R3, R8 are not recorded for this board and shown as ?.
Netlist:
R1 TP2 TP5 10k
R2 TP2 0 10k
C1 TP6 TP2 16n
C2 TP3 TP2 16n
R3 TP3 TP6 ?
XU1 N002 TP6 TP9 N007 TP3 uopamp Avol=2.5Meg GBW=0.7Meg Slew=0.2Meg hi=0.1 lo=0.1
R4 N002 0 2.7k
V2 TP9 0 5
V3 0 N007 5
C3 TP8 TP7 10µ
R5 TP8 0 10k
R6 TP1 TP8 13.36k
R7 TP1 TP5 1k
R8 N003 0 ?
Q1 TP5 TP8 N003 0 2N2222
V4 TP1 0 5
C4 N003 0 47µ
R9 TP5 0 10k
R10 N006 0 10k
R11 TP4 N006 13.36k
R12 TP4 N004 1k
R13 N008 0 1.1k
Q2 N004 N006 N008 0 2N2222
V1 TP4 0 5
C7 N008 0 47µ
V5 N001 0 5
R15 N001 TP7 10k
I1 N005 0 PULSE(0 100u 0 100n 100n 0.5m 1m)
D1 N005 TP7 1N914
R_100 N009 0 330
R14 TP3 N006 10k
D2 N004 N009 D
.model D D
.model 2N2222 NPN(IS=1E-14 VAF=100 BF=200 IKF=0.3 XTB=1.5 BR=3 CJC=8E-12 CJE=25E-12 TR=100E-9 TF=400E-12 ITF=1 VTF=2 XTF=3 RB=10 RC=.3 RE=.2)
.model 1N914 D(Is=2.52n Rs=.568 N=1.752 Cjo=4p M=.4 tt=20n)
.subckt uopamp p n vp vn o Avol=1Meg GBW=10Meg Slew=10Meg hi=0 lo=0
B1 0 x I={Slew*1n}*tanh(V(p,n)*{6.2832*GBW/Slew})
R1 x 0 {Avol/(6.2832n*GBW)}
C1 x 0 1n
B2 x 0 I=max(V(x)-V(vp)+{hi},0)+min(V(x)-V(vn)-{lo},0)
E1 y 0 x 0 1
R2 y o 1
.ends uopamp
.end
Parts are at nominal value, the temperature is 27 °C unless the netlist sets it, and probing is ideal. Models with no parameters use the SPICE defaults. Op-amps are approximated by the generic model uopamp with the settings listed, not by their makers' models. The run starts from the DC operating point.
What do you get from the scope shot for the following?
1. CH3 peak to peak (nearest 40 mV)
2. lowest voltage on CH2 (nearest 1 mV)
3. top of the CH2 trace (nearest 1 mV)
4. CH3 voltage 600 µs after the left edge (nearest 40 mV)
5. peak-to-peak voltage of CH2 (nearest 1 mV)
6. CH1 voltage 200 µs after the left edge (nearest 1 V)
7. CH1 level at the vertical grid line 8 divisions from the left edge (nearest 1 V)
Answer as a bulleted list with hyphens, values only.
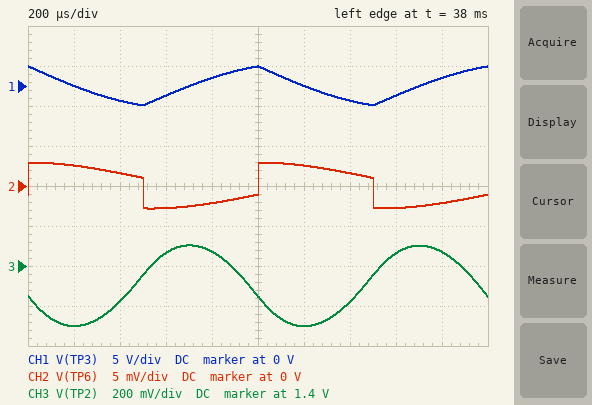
- 400 mV
- -3 mV
- 3 mV
- 1.48 V
- 6 mV
- 0 V
- -1 V
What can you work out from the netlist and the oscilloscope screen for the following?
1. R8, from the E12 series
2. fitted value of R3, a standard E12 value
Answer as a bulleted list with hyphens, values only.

- 560 Ω
- 100 kΩ
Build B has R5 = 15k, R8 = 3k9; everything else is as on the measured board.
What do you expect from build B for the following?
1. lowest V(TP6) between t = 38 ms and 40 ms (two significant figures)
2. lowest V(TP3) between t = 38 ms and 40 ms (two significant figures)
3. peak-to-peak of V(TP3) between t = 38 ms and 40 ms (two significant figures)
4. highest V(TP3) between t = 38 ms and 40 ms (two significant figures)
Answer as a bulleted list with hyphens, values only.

- -1.0 mV
- -830 mV
- 1.6 V
- 800 mV
